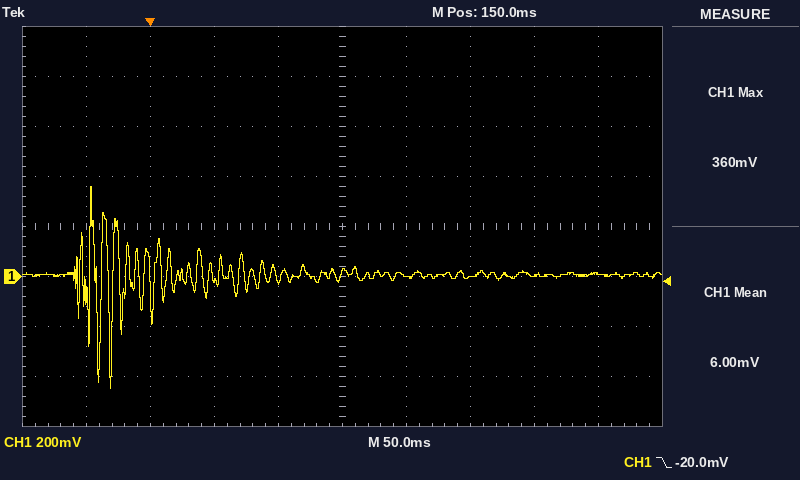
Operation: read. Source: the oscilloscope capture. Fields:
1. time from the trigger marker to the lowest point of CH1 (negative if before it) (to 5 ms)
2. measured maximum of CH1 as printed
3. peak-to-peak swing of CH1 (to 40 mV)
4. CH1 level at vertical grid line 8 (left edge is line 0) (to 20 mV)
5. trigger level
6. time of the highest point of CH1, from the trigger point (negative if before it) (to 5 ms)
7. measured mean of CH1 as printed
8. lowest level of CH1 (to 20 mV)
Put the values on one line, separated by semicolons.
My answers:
-30 ms; 360 mV; 800 mV; 0 mV; -20.0 mV; -45 ms; 6.00 mV; -440 mV
